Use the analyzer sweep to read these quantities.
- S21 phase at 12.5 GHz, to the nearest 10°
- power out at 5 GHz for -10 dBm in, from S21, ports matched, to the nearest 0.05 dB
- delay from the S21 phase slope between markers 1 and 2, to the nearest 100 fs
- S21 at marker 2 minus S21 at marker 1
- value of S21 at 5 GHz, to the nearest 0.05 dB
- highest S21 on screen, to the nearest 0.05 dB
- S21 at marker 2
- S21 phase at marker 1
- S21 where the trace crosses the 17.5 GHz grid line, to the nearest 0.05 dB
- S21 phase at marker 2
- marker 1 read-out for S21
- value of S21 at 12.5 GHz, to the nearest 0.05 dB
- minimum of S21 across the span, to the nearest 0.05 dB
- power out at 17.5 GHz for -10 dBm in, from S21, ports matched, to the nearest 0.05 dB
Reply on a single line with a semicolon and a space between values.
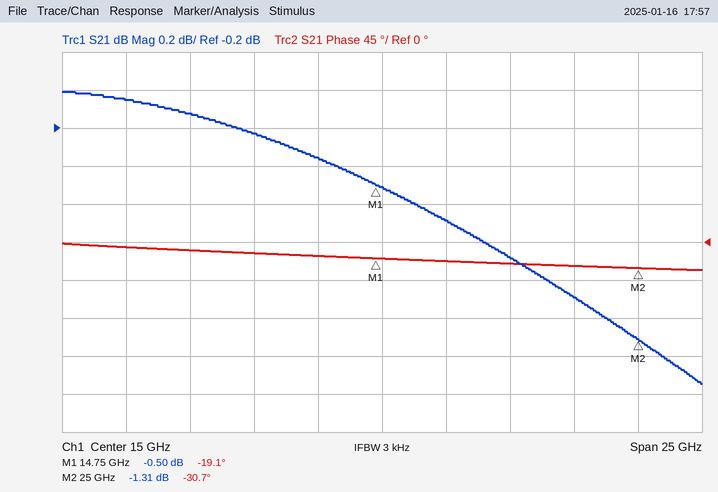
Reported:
-20°; -10.05 dBm; 3.1 ps; -0.81 dB; -0.05 dB; 0.00 dB; -1.31 dB; -19.1°; -0.70 dB; -30.7°; -0.50 dB; -0.35 dB; -1.55 dB; -10.70 dBm
